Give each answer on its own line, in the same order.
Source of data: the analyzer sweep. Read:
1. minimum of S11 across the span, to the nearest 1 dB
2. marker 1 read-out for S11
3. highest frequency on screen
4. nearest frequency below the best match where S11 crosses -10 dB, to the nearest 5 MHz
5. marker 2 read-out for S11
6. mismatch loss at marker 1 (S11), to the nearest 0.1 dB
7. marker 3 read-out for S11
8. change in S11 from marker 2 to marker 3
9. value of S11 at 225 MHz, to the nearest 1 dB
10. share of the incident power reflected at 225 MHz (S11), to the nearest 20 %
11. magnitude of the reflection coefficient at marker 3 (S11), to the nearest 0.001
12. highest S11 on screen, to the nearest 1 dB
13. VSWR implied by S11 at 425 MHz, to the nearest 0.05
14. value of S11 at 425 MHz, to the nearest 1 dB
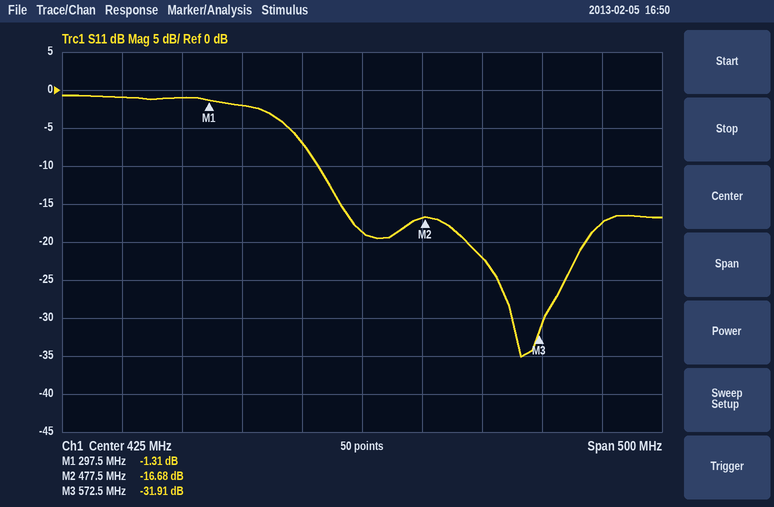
-35 dB
-1.31 dB
675 MHz
390 MHz
-16.68 dB
5.8 dB
-31.91 dB
-15.23 dB
-1 dB
80 %
0.025
-1 dB
1.25
-19 dB
